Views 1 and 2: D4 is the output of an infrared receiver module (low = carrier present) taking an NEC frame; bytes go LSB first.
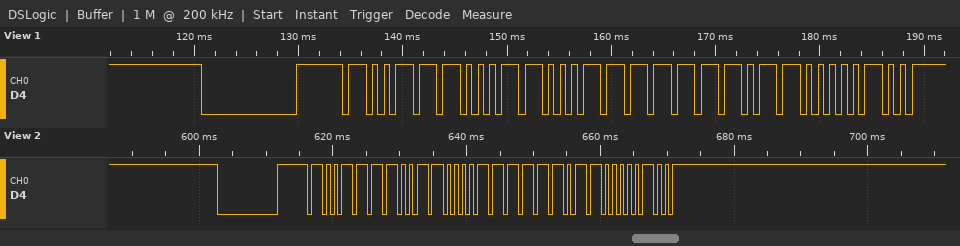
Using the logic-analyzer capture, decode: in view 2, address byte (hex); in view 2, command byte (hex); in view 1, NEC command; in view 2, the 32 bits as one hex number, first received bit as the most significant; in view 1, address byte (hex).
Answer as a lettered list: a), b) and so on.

a) 0x79
b) 0xDF
c) 0xDF
d) 0x9E61FB04
e) 0x39
